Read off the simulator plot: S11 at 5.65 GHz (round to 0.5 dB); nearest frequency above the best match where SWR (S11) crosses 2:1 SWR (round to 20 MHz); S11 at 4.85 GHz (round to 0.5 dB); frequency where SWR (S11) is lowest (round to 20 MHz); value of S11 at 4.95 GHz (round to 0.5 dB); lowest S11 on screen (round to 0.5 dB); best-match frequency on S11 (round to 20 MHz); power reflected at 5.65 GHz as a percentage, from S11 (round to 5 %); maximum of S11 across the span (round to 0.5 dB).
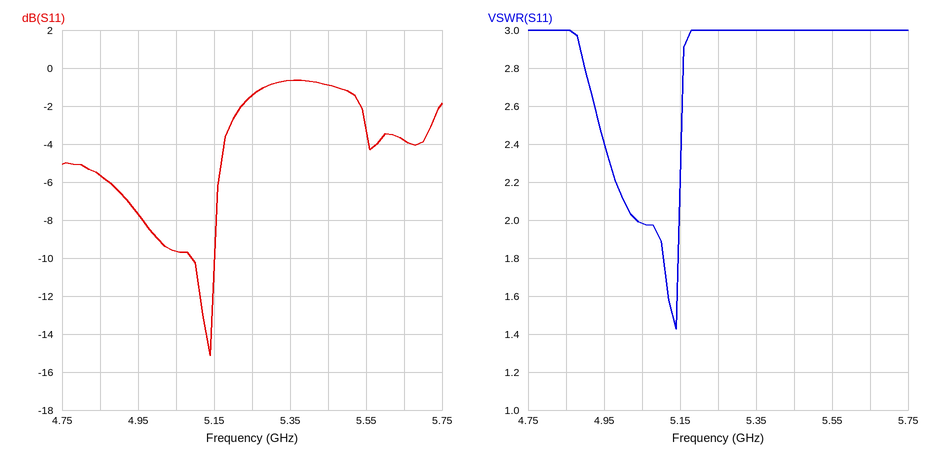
-4.0 dB
5.14 GHz
-5.5 dB
5.14 GHz
-7.5 dB
-15.0 dB
5.14 GHz
40 %
-0.5 dB
